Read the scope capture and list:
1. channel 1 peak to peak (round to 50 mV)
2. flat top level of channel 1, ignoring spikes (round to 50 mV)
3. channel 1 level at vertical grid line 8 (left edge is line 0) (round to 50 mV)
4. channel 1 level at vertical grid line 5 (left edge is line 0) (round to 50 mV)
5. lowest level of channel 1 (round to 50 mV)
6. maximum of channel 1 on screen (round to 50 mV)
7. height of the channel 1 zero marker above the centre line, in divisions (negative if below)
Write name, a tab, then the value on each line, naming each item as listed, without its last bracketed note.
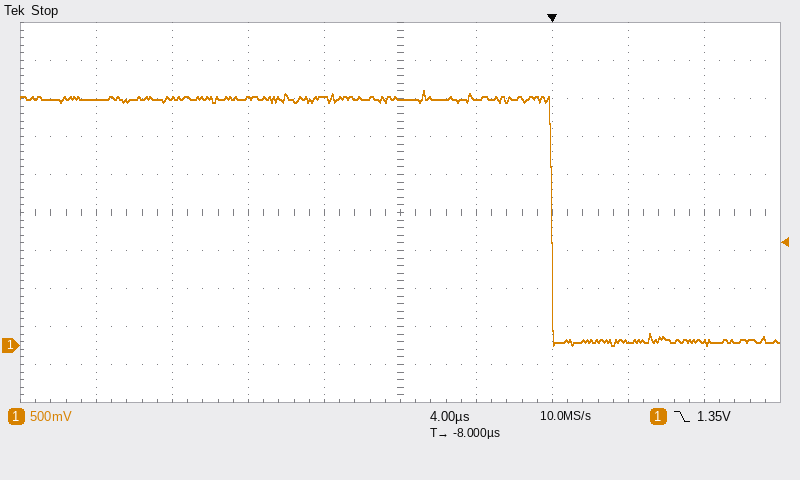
channel 1 peak to peak	3.35 V
flat top level of channel 1, ignoring spikes	3.25 V
channel 1 level at vertical grid line 8 (left edge is line 0)	50 mV
channel 1 level at vertical grid line 5 (left edge is line 0)	3.25 V
lowest level of channel 1	0 mV
maximum of channel 1 on screen	3.35 V
height of the channel 1 zero marker above the centre line, in divisions	-3.5 div
